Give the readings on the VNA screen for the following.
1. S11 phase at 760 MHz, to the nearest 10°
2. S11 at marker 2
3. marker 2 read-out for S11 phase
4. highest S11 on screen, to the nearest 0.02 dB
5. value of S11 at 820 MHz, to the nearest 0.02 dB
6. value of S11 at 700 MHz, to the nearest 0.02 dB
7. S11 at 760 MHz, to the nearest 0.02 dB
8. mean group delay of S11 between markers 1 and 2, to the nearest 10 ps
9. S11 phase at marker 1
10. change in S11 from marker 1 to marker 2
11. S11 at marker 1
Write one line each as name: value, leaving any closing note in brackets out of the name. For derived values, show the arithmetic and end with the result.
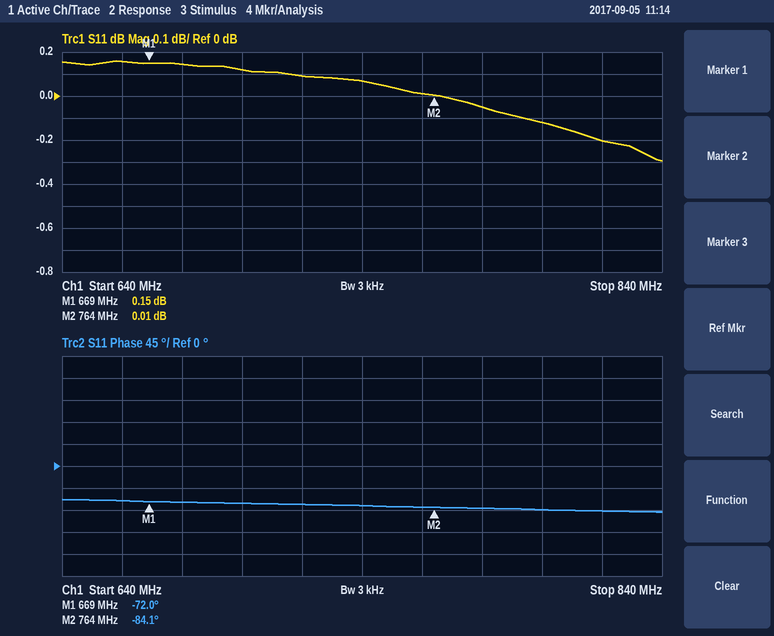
S11 phase at 760 MHz, to the nearest 10°: -80°
S11 at marker 2: 0.01 dB
marker 2 read-out for S11 phase: -84.1°
highest S11 on screen, to the nearest 0.02 dB: 0.16 dB
value of S11 at 820 MHz, to the nearest 0.02 dB: -0.20 dB
value of S11 at 700 MHz, to the nearest 0.02 dB: 0.12 dB
S11 at 760 MHz, to the nearest 0.02 dB: 0.02 dB
mean group delay of S11 between markers 1 and 2, to the nearest 10 ps: −(-84.1° − (-72°))/(360° × 95 MHz) ≈ 354 ps, so 350 ps to the nearest 10 ps
S11 phase at marker 1: -72.0°
change in S11 from marker 1 to marker 2: 0.01 − (0.15) = -0.14 dB
S11 at marker 1: 0.15 dB
